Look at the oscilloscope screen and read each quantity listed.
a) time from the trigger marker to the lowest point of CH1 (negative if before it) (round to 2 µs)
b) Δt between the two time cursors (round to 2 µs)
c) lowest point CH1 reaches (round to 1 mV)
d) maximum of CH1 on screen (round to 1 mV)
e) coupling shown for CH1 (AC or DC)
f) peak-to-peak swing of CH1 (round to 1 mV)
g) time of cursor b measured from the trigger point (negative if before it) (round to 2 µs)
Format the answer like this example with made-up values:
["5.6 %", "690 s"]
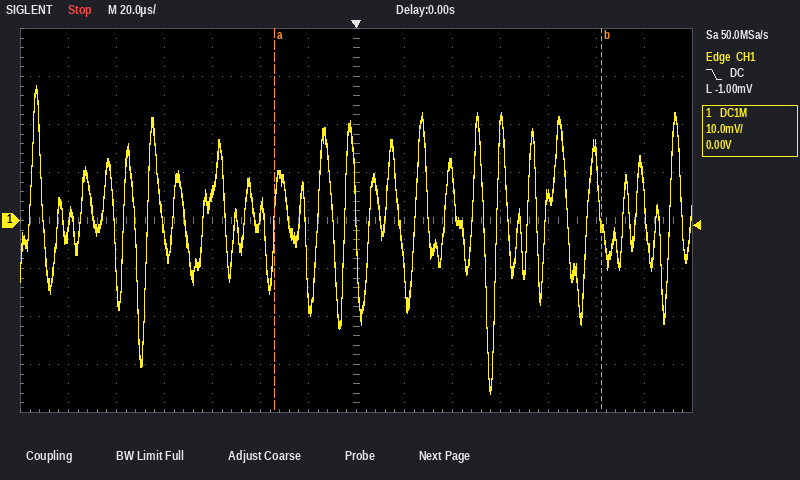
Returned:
["+56 µs", "136 µs", "-36 mV", "28 mV", "DC", "64 mV", "+102 µs"]
